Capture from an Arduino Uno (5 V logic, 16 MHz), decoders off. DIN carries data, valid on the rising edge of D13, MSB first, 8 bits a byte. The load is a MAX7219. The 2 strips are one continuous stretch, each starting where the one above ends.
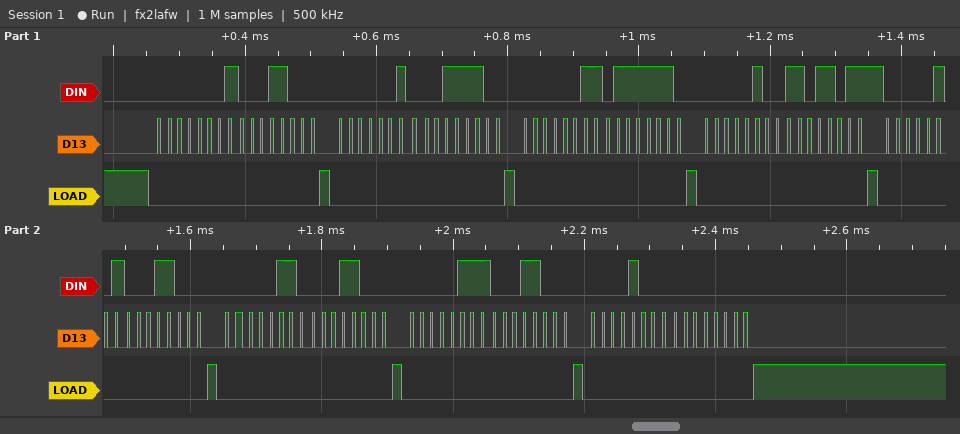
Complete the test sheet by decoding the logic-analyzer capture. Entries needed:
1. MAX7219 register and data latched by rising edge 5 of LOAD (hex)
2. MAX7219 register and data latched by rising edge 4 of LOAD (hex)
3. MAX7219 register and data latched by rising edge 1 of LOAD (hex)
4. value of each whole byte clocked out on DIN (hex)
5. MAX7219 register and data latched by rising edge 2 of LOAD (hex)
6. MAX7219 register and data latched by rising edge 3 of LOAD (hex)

register 0x5, data 0x18
register 0x4, data 0xDB
register 0x1, data 0x18
01 18 02 3C 03 7E 04 DB 05 18 06 18 07 18 08 00
register 0x2, data 0x3C
register 0x3, data 0x7E
